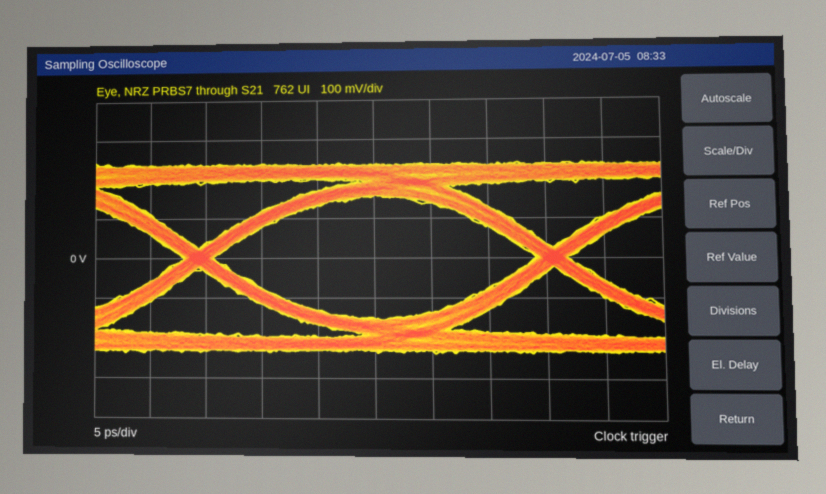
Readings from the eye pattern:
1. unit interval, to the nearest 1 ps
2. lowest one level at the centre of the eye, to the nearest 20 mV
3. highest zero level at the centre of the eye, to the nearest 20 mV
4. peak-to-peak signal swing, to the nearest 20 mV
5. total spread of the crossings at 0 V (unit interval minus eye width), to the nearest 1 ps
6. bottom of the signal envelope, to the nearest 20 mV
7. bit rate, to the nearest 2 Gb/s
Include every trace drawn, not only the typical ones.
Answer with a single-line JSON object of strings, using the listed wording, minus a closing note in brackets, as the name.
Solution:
{"unit interval, to the nearest 1 ps": "31 ps", "lowest one level at the centre of the eye, to the nearest 20 mV": "160 mV", "highest zero level at the centre of the eye, to the nearest 20 mV": "-160 mV", "peak-to-peak signal swing, to the nearest 20 mV": "480 mV", "total spread of the crossings at 0 V (unit interval minus eye width), to the nearest 1 ps": "3 ps", "bottom of the signal envelope, to the nearest 20 mV": "-240 mV", "bit rate, to the nearest 2 Gb/s": "32 Gb/s"}
